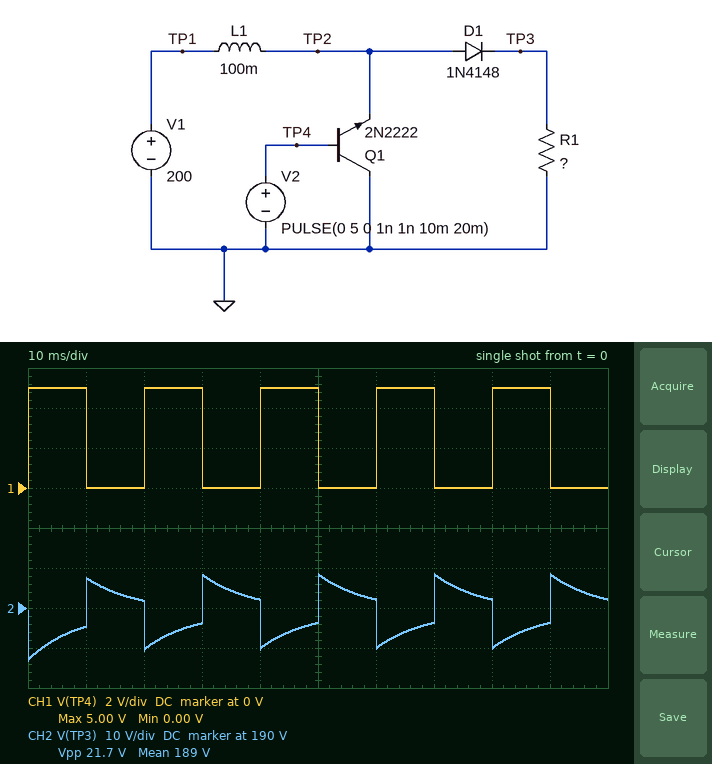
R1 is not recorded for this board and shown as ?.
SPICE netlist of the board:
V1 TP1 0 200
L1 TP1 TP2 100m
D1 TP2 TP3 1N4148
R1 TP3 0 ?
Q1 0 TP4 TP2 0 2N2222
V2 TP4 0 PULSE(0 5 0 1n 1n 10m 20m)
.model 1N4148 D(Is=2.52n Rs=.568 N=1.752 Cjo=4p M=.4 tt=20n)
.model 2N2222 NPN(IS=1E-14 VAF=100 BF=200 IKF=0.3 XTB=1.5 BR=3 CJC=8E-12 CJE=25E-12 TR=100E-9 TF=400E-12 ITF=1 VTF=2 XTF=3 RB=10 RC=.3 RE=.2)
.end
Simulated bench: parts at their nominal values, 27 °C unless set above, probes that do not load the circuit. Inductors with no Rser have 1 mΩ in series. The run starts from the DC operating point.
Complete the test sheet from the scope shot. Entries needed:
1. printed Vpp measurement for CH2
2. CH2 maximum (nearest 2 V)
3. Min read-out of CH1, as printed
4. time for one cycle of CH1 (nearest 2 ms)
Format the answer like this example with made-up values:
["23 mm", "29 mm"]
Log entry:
["21.7 V", "198 V", "0.00 V", "20 ms"]
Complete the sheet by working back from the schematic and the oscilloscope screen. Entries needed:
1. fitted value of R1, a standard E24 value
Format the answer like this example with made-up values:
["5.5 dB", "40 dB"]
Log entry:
["11 Ω"]
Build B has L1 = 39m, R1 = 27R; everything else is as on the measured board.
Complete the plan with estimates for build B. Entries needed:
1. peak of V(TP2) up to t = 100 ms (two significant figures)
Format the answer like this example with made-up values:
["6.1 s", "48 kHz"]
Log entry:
["230 V"]
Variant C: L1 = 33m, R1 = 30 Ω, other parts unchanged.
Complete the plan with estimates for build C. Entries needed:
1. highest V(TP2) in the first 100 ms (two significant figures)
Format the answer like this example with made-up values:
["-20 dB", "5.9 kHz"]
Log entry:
["230 V"]
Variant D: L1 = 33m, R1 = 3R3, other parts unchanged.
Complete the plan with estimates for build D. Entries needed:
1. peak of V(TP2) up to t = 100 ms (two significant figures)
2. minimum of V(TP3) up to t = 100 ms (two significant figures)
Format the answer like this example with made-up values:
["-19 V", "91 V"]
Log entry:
["200 V", "170 V"]
